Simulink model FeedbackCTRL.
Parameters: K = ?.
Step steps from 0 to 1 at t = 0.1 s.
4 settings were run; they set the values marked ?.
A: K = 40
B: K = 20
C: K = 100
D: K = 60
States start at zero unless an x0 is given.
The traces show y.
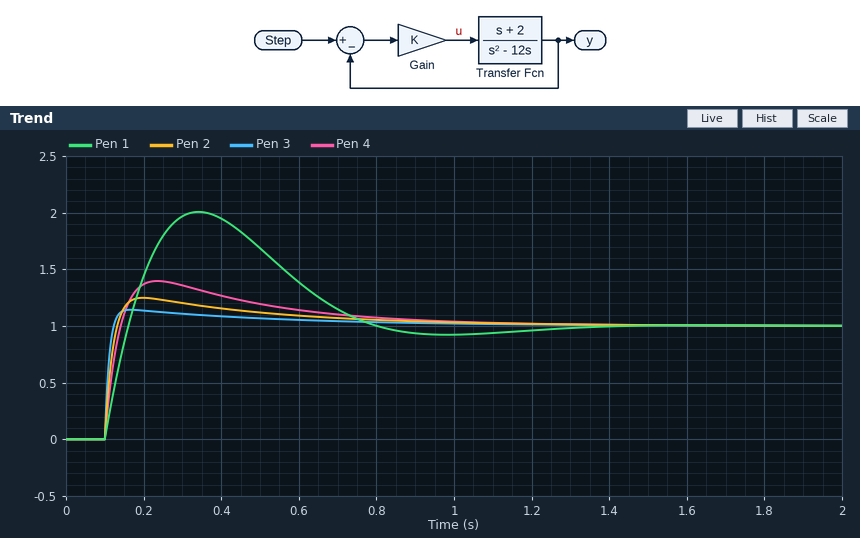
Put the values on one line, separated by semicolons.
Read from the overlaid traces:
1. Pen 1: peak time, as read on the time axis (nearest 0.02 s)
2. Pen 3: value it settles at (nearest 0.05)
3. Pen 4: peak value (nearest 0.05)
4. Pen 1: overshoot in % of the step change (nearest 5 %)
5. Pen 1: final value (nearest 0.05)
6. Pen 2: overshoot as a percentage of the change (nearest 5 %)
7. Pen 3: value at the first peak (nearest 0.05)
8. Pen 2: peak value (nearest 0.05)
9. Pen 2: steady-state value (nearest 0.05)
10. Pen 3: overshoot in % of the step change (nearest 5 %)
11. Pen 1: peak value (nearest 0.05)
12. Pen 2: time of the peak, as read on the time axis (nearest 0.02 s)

0.34 s; 1.00; 1.40; 100 %; 1.00; 25 %; 1.15; 1.25; 1.00; 15 %; 2.00; 0.20 s
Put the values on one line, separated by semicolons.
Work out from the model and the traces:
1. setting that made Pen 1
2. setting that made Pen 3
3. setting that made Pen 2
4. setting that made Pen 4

B; C; D; A
